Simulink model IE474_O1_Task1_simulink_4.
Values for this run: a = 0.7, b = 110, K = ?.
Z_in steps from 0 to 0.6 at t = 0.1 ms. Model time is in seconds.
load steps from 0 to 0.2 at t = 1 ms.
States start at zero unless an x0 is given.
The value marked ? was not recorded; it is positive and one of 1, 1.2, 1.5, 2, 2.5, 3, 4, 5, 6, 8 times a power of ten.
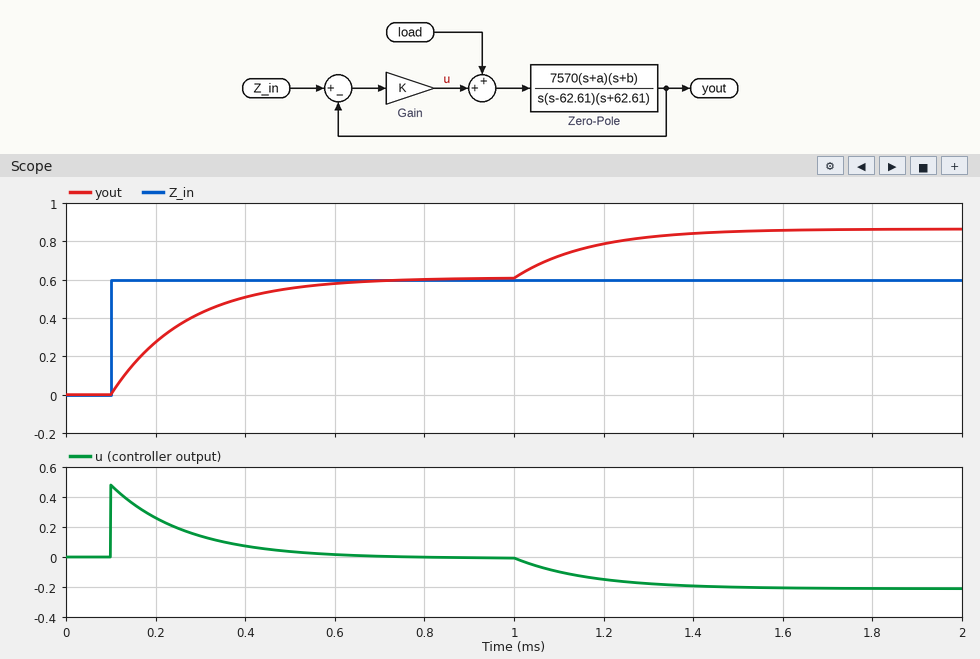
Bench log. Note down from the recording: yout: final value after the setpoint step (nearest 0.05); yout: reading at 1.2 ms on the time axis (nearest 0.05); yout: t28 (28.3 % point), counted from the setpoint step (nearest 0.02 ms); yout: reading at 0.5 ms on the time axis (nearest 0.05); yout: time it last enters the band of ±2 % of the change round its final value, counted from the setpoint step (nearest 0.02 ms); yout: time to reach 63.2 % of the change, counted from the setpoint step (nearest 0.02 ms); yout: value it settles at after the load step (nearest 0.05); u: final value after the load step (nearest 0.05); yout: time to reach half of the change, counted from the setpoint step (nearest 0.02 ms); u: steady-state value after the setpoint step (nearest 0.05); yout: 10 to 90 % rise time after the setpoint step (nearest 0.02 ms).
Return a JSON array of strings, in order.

["0.60", "0.80", "0.06 ms", "0.55", "0.60 ms", "0.16 ms", "0.85", "-0.20", "0.12 ms", "0.00", "0.36 ms"]
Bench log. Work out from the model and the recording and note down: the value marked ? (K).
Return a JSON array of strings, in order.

["0.8"]
